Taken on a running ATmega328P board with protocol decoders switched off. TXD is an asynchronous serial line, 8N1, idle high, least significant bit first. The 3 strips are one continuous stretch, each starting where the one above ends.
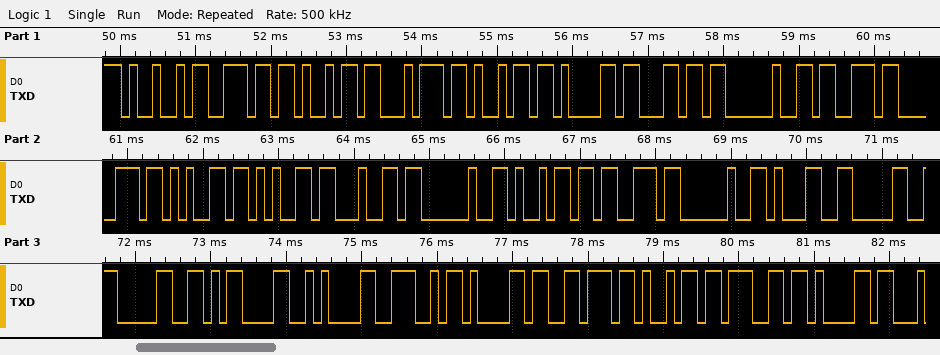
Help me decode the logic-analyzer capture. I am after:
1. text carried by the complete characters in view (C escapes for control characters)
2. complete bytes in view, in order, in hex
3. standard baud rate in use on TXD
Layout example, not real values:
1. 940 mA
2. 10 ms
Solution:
1. "Initial speed is 100\r\nNaviga"
2. 0x49 0x6E 0x69 0x74 0x69 0x61 0x6C 0x20 0x73 0x70 0x65 0x65 0x64 0x20 0x69 0x73 0x20 0x31 0x30 0x30 0x0D 0x0A 0x4E 0x61 0x76 0x69 0x67 0x61
3. 9600 baud
